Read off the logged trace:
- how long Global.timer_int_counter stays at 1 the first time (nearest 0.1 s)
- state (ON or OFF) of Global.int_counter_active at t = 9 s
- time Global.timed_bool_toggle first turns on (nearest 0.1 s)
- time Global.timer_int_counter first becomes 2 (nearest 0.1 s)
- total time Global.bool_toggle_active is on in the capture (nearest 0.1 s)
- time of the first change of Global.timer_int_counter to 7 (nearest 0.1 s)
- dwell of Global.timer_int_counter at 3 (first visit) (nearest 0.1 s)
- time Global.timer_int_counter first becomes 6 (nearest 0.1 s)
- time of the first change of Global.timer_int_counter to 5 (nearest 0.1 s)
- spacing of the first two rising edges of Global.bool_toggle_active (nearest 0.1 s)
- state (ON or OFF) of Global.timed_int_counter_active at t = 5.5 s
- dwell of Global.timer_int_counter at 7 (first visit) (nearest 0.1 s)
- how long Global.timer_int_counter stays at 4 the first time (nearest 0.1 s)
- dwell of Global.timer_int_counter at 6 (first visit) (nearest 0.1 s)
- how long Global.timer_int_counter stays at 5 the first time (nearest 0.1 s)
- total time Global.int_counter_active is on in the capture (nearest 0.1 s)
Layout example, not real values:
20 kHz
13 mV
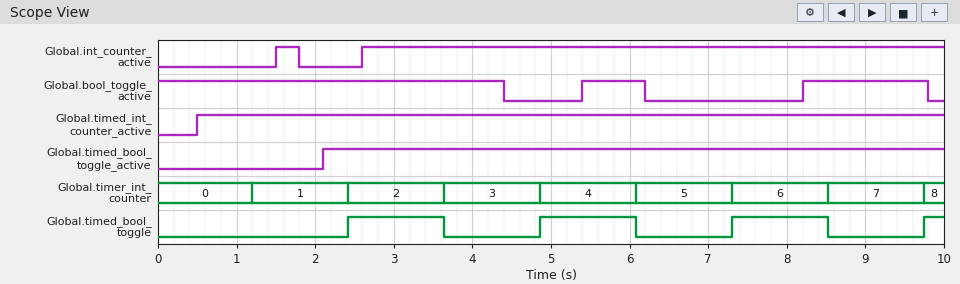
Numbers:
1.2 s
ON
2.4 s
2.4 s
6.8 s
8.5 s
1.2 s
7.3 s
6.1 s
2.8 s
ON
1.2 s
1.2 s
1.2 s
1.2 s
7.7 s
